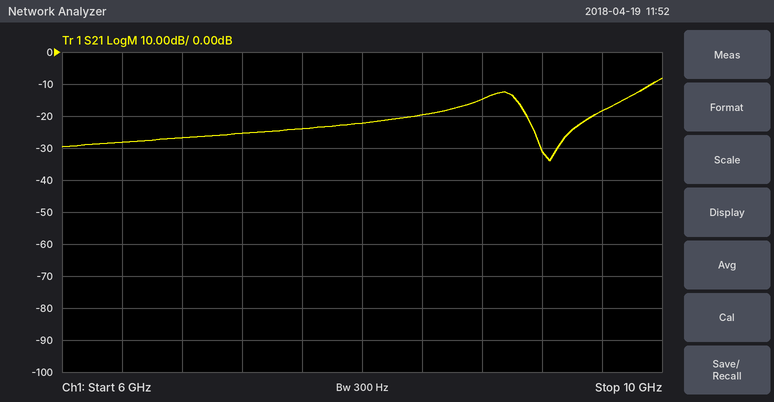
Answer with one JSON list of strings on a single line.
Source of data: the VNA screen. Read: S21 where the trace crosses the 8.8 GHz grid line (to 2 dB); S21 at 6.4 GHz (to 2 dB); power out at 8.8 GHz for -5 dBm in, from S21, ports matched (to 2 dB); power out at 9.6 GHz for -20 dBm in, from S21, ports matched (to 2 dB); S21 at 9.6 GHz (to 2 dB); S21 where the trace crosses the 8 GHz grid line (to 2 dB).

["-14 dB", "-28 dB", "-20 dBm", "-38 dBm", "-18 dB", "-22 dB"]
